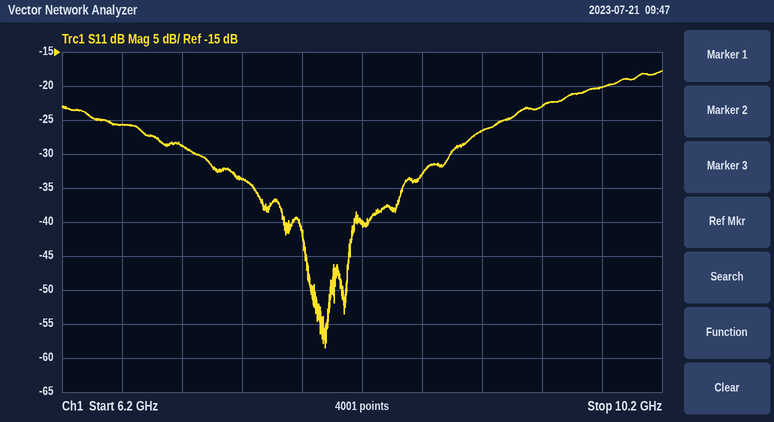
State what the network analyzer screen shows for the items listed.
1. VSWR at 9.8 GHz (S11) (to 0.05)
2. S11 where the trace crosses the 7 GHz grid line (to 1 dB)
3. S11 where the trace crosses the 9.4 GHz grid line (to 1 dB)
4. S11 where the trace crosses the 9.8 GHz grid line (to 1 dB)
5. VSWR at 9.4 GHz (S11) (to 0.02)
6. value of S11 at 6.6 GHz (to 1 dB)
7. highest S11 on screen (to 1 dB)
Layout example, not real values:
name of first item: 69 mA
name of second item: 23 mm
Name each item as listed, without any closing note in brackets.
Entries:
VSWR at 9.8 GHz (S11): 1.20
S11 where the trace crosses the 7 GHz grid line: -29 dB
S11 where the trace crosses the 9.4 GHz grid line: -23 dB
S11 where the trace crosses the 9.8 GHz grid line: -20 dB
VSWR at 9.4 GHz (S11): 1.16
value of S11 at 6.6 GHz: -26 dB
highest S11 on screen: -18 dB
